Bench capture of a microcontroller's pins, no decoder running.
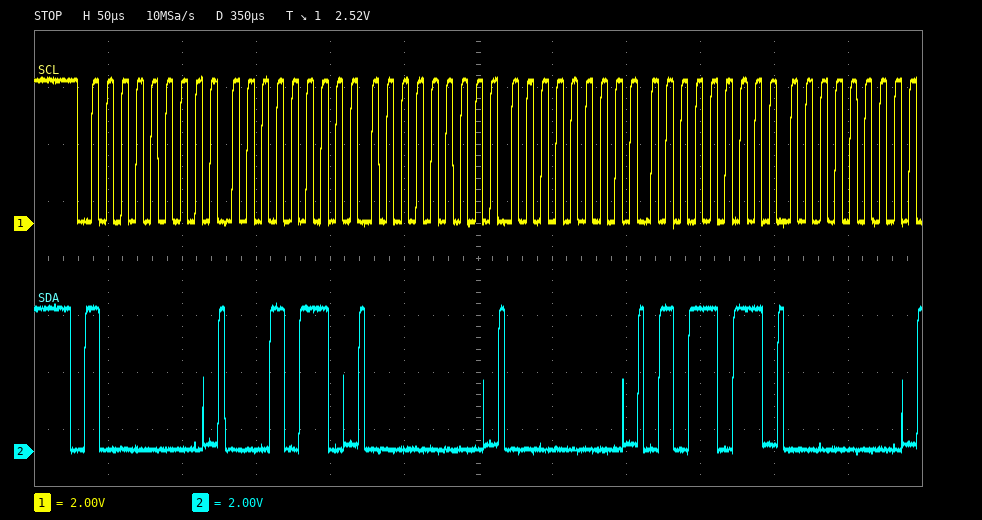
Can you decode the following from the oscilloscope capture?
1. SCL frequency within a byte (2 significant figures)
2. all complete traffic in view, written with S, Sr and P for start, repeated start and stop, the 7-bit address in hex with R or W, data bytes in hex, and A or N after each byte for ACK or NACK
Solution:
100 kHz
S 40W A 16 A 00 A 00 A 5B A 00 A
